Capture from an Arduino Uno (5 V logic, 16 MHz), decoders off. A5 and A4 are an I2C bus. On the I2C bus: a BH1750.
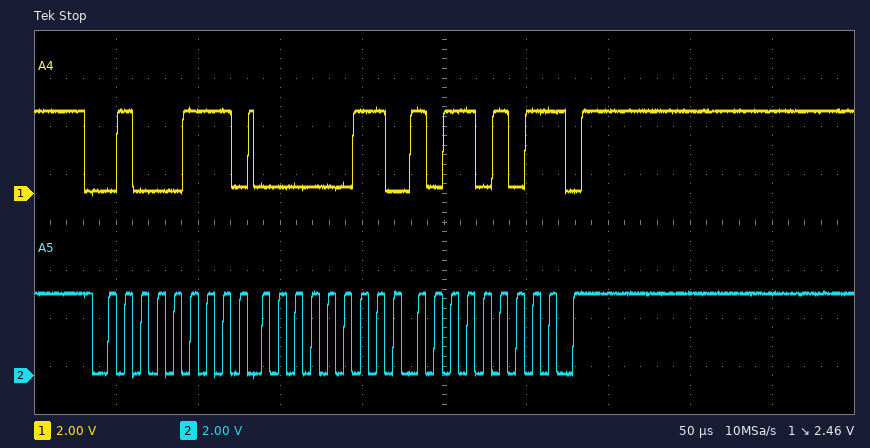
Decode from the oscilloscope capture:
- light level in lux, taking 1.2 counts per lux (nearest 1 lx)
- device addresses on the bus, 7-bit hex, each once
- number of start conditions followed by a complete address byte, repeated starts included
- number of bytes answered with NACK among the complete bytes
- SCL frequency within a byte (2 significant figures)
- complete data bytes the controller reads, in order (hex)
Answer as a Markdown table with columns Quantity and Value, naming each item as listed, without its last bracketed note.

| Quantity | Value |
|---|---|
| light level in lux, taking 1.2 counts per lux | 791 lx |
| device addresses on the bus, 7-bit hex, each once | 0x23 |
| number of start conditions followed by a complete address byte, repeated starts included | 1 |
| number of bytes answered with NACK among the complete bytes | 1 |
| SCL frequency within a byte | 100 kHz |
| complete data bytes the controller reads, in order | 03 B5 |
